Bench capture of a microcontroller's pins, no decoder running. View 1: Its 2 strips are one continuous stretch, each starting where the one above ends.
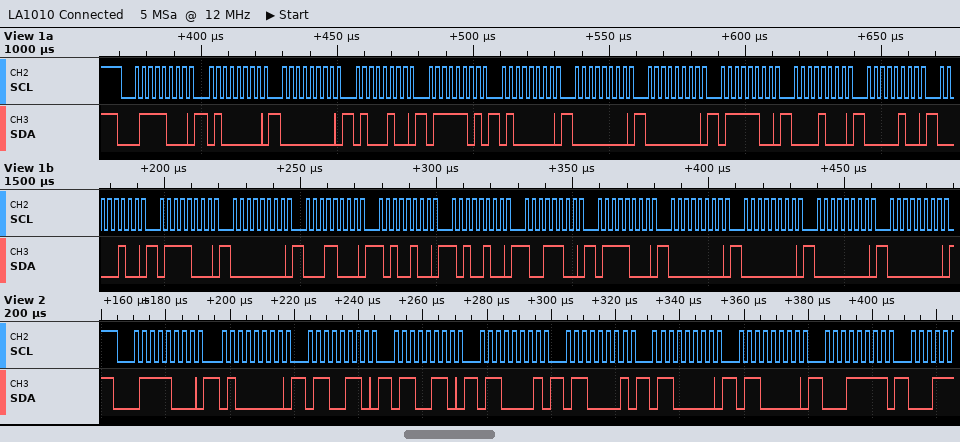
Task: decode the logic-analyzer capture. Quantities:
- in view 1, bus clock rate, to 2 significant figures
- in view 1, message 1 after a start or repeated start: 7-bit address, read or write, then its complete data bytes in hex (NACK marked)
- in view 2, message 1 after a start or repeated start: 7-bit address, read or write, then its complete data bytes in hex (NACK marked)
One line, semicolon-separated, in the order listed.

400 kHz; 0x3C write: 40 00 44 7D 40 00 00 7C 08 04 04 78 00 18 A4 A4 9C 78 00 00 00 00; 0x3C write: 40 66 66 61 61 60 60 1F
